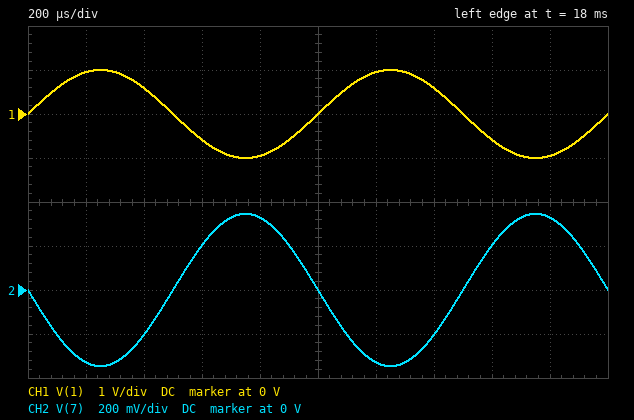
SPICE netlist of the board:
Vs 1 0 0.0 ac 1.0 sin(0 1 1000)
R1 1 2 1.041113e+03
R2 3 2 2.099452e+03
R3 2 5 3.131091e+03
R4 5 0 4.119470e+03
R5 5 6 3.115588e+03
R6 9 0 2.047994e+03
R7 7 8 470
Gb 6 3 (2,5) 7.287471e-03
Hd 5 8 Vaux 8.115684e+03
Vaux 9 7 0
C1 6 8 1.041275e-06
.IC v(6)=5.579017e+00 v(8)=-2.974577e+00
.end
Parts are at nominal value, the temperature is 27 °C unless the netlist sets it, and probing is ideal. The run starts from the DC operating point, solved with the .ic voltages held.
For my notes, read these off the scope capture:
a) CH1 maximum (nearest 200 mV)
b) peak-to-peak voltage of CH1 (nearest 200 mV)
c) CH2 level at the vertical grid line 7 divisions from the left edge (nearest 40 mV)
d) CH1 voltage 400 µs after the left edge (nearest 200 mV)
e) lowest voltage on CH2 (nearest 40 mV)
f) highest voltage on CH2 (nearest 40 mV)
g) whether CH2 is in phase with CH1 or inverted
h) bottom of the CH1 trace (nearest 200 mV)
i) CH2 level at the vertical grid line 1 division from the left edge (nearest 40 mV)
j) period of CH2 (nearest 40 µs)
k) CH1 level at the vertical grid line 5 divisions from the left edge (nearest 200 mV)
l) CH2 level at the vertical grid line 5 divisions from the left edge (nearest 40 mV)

1.0 V
2.0 V
-200 mV
600 mV
-360 mV
360 mV
inverted
-1.0 V
-320 mV
1.00 ms
0 V
0 V
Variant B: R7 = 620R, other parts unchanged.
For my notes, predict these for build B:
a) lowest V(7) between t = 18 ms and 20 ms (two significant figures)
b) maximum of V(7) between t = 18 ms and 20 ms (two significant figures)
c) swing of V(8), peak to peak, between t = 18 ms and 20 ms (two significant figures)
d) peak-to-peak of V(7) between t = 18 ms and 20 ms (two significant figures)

-360 mV
360 mV
930 mV
710 mV
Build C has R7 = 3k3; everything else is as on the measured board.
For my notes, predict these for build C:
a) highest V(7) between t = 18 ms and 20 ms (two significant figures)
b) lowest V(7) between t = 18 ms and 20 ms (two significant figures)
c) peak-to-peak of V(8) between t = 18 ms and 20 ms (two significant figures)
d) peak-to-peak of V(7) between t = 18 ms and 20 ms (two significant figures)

830 mV
-830 mV
4.3 V
1.7 V
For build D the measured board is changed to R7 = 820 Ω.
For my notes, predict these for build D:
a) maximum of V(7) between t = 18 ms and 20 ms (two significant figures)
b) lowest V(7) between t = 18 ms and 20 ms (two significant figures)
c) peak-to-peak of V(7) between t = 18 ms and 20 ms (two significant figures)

370 mV
-370 mV
750 mV
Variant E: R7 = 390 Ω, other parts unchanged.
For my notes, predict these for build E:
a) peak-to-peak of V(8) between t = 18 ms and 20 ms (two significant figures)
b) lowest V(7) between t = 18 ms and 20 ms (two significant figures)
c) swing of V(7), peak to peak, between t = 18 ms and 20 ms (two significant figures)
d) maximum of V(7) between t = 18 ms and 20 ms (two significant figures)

810 mV
-340 mV
680 mV
340 mV
